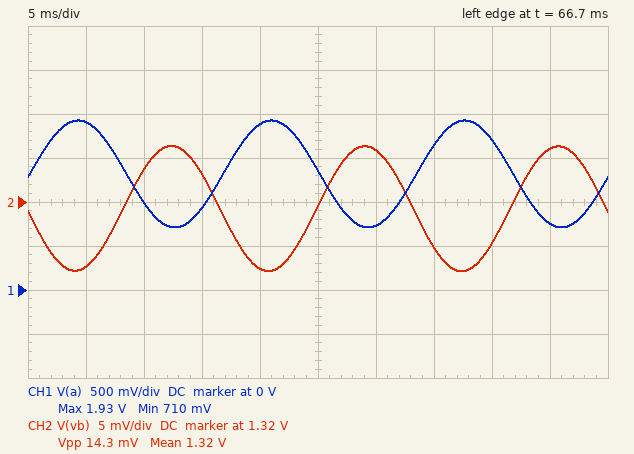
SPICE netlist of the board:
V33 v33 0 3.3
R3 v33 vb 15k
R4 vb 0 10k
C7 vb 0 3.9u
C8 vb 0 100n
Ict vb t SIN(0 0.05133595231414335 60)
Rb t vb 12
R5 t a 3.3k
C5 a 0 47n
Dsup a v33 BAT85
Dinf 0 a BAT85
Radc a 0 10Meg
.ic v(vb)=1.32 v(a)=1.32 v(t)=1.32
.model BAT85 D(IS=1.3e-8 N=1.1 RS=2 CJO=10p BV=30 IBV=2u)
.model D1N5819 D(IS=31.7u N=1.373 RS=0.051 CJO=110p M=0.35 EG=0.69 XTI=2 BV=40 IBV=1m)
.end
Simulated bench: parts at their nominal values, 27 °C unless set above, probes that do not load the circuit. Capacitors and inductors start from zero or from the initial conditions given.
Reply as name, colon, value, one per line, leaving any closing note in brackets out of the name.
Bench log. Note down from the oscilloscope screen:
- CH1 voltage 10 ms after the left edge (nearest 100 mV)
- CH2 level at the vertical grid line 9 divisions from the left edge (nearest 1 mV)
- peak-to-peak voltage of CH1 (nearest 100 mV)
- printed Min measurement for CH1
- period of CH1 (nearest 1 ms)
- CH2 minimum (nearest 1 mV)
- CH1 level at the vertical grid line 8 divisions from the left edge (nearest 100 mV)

CH1 voltage 10 ms after the left edge: 1.0 V
CH2 level at the vertical grid line 9 divisions from the left edge: 1.326 V
peak-to-peak voltage of CH1: 1.2 V
printed Min measurement for CH1: 710 mV
period of CH1: 17 ms
CH2 minimum: 1.312 V
CH1 level at the vertical grid line 8 divisions from the left edge: 1.7 V
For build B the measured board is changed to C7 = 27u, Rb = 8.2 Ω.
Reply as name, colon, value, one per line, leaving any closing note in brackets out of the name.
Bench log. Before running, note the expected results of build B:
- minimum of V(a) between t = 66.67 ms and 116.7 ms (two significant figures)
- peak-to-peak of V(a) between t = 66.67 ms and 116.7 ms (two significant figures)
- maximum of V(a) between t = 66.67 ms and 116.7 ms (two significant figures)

minimum of V(a) between t = 66.67 ms and 116.7 ms: 900 mV
peak-to-peak of V(a) between t = 66.67 ms and 116.7 ms: 840 mV
maximum of V(a) between t = 66.67 ms and 116.7 ms: 1.7 V
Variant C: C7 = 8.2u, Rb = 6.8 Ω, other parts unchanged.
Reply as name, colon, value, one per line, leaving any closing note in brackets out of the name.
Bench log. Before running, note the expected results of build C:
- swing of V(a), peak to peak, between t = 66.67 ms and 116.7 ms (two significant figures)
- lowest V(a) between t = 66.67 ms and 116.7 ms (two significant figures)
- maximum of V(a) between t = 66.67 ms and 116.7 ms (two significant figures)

swing of V(a), peak to peak, between t = 66.67 ms and 116.7 ms: 690 mV
lowest V(a) between t = 66.67 ms and 116.7 ms: 970 mV
maximum of V(a) between t = 66.67 ms and 116.7 ms: 1.7 V
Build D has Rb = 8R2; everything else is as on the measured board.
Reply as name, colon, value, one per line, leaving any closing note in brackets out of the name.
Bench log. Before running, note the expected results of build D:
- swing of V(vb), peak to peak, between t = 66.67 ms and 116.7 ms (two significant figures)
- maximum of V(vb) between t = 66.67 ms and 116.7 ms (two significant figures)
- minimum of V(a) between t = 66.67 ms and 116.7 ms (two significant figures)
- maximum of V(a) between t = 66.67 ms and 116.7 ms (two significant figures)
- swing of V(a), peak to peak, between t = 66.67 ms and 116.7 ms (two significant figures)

swing of V(vb), peak to peak, between t = 66.67 ms and 116.7 ms: 9.7 mV
maximum of V(vb) between t = 66.67 ms and 116.7 ms: 1.3 V
minimum of V(a) between t = 66.67 ms and 116.7 ms: 900 mV
maximum of V(a) between t = 66.67 ms and 116.7 ms: 1.7 V
swing of V(a), peak to peak, between t = 66.67 ms and 116.7 ms: 830 mV
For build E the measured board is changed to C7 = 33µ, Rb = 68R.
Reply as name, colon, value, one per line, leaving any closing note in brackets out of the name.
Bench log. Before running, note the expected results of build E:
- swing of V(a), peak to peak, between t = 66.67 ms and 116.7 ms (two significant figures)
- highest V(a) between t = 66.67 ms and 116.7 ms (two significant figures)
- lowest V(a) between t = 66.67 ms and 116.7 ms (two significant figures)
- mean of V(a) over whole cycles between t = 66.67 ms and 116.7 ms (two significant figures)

swing of V(a), peak to peak, between t = 66.67 ms and 116.7 ms: 3.9 V
highest V(a) between t = 66.67 ms and 116.7 ms: 3.6 V
lowest V(a) between t = 66.67 ms and 116.7 ms: -300 mV
mean of V(a) over whole cycles between t = 66.67 ms and 116.7 ms: 1.6 V
